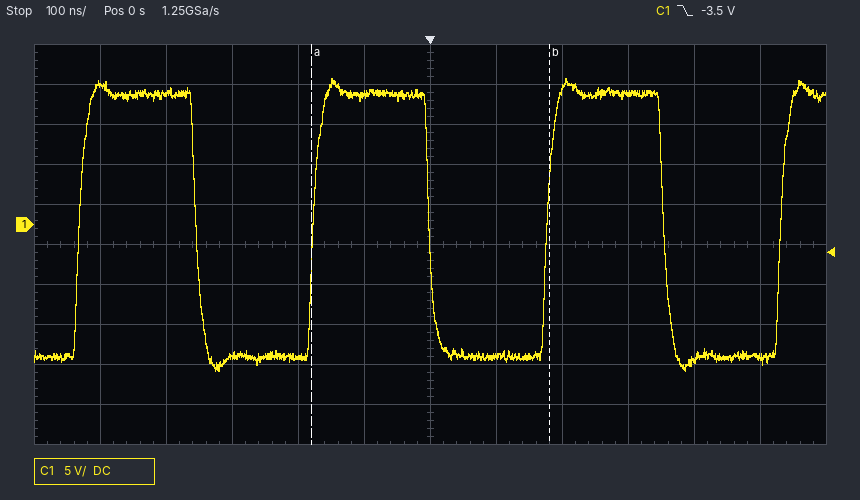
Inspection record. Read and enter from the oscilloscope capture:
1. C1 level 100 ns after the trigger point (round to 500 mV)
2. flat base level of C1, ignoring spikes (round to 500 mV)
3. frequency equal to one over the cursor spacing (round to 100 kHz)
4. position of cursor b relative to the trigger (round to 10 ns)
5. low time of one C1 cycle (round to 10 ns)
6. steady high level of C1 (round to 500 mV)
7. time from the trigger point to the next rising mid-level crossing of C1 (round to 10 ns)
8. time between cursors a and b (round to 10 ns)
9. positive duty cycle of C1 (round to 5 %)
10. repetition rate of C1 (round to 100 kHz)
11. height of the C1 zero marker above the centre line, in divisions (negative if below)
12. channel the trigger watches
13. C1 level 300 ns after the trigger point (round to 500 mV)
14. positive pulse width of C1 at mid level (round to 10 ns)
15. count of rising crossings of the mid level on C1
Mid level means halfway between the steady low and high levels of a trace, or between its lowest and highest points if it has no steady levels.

-16.5 V
-16.5 V
2.8 MHz
+180 ns
180 ns
16.5 V
180 ns
360 ns
50 %
2.8 MHz
+0.5 div
C1
16.5 V
180 ns
4
